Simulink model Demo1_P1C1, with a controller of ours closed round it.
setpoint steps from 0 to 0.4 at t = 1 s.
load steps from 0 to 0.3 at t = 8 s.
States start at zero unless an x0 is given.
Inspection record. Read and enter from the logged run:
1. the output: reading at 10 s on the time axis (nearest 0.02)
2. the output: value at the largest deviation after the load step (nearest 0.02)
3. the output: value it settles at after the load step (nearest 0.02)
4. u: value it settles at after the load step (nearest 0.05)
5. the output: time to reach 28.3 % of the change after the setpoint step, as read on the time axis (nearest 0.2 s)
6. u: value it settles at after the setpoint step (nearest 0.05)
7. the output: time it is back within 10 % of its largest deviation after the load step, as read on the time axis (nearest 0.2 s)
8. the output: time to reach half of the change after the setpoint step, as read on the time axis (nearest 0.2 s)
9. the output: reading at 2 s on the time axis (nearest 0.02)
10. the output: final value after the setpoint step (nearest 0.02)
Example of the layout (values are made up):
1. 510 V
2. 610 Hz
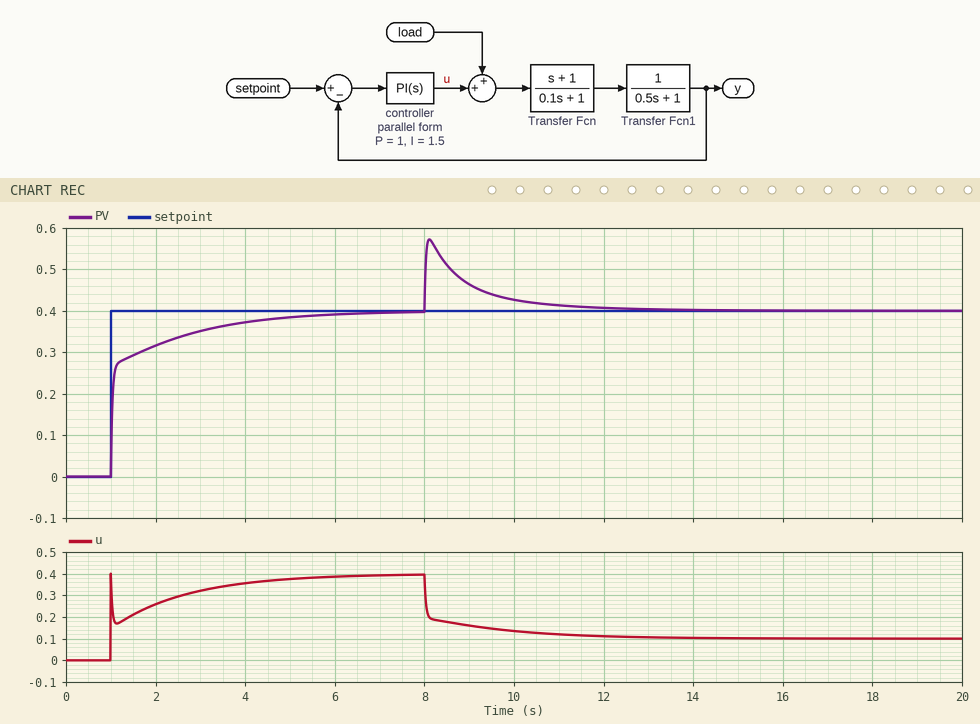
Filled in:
1. 0.42
2. 0.58
3. 0.40
4. 0.10
5. 1.0 s
6. 0.40
7. 10.6 s
8. 1.0 s
9. 0.32
10. 0.40
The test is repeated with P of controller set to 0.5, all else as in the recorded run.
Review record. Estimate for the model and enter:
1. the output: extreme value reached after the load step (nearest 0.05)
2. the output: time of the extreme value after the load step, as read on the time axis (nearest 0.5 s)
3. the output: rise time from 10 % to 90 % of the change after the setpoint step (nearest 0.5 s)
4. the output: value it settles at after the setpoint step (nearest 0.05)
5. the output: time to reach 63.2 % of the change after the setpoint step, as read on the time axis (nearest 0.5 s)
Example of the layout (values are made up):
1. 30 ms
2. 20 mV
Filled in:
1. 0.65
2. 8.0 s
3. 2.0 s
4. 0.40
5. 1.5 s
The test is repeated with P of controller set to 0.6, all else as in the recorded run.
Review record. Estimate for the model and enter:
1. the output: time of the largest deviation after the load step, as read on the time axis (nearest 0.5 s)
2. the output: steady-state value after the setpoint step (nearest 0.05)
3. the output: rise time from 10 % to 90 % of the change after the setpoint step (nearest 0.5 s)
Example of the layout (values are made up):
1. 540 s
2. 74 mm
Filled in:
1. 8.0 s
2. 0.40
3. 2.0 s
